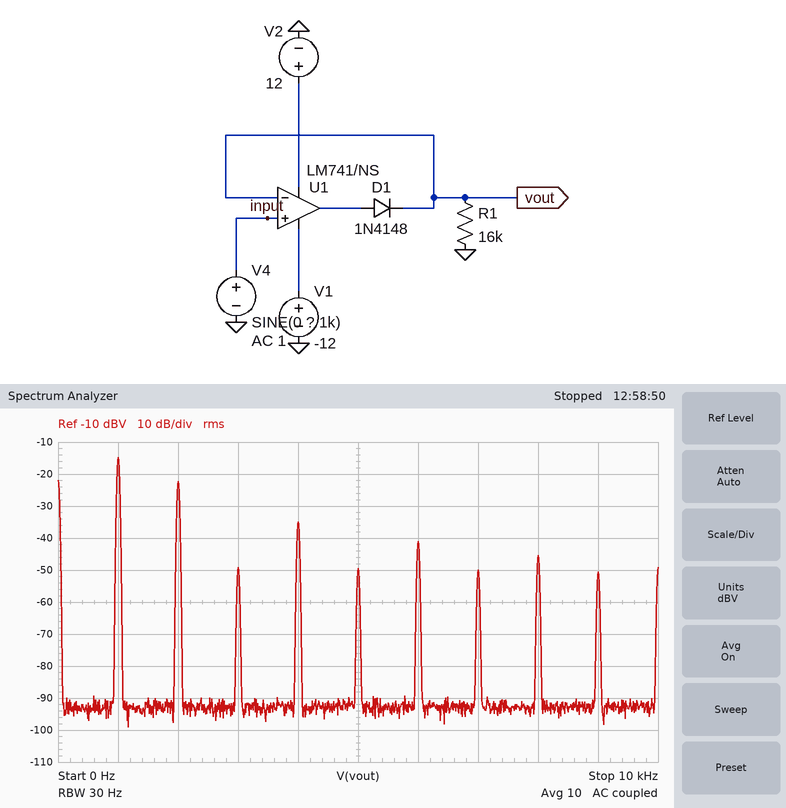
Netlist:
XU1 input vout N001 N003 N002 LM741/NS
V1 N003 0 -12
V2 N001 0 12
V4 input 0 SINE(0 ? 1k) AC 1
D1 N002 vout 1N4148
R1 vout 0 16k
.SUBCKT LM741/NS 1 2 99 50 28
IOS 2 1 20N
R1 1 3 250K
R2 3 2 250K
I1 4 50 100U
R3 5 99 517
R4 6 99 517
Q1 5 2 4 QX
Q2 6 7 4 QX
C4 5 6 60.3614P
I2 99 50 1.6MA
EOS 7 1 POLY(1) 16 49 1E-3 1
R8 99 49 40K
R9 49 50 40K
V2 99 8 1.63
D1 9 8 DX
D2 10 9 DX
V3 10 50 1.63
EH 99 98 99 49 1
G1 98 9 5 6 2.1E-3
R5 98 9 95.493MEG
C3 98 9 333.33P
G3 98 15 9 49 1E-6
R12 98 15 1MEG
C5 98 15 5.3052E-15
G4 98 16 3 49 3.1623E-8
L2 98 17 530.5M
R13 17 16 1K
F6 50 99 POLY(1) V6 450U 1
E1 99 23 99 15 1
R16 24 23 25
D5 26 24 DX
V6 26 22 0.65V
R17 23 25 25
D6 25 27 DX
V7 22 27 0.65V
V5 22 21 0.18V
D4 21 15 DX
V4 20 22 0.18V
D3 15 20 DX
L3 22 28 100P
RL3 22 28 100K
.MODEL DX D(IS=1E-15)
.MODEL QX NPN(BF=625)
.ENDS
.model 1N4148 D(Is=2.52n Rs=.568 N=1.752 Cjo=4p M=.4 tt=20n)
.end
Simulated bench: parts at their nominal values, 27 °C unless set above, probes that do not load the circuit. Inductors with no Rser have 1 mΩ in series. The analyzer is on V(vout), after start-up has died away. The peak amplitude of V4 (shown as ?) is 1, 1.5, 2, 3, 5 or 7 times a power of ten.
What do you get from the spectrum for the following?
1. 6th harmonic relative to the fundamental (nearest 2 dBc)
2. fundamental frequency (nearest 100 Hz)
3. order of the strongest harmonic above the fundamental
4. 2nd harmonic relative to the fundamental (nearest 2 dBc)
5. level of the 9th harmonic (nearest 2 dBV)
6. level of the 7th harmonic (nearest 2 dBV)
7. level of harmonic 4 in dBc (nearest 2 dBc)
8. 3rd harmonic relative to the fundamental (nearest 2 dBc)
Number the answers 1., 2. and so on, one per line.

1. -26 dBc
2. 1.0 kHz
3. 2
4. -8 dBc
5. -50 dBV
6. -50 dBV
7. -20 dBc
8. -34 dBc
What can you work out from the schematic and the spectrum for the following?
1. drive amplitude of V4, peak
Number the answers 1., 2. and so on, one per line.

1. 500 mV
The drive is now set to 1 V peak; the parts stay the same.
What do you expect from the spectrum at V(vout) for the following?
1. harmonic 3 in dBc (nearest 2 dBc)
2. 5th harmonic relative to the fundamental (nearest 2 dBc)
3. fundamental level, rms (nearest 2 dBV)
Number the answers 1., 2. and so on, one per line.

1. -36 dBc
2. -36 dBc
3. -8 dBV
